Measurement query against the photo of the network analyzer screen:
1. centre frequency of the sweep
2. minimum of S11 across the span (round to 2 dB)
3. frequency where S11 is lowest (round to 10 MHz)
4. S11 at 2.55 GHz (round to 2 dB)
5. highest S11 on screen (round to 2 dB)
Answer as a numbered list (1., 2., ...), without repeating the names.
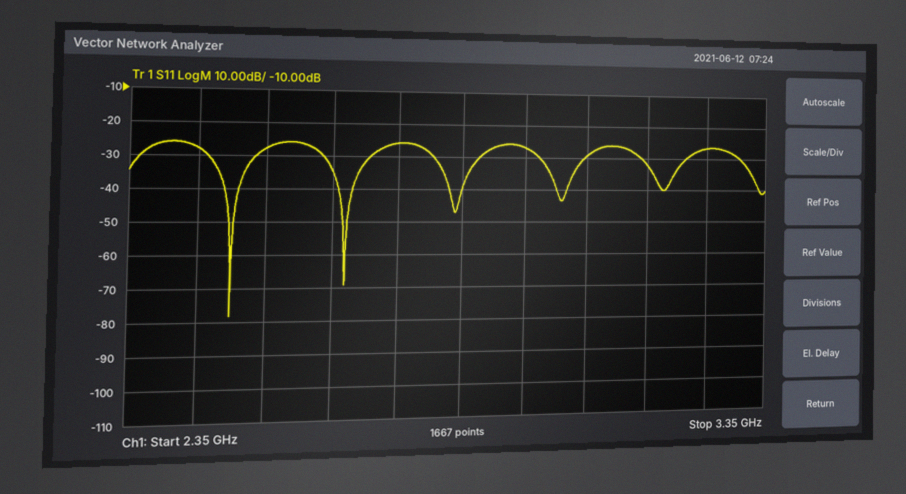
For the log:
1. 2.85 GHz
2. -78 dB
3. 2.50 GHz
4. -28 dB
5. -26 dB
